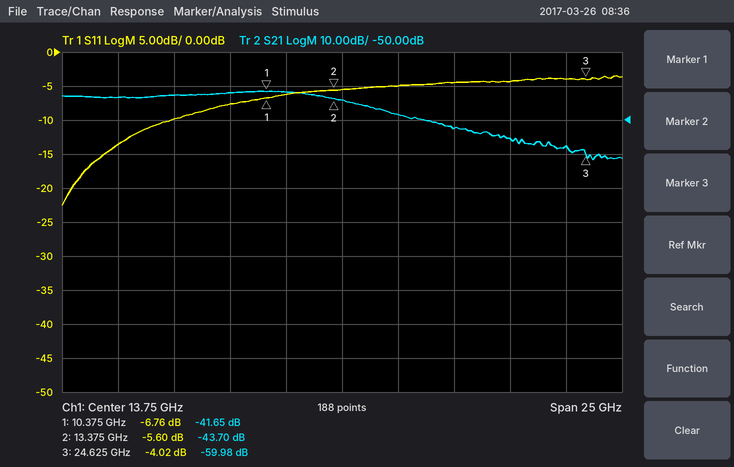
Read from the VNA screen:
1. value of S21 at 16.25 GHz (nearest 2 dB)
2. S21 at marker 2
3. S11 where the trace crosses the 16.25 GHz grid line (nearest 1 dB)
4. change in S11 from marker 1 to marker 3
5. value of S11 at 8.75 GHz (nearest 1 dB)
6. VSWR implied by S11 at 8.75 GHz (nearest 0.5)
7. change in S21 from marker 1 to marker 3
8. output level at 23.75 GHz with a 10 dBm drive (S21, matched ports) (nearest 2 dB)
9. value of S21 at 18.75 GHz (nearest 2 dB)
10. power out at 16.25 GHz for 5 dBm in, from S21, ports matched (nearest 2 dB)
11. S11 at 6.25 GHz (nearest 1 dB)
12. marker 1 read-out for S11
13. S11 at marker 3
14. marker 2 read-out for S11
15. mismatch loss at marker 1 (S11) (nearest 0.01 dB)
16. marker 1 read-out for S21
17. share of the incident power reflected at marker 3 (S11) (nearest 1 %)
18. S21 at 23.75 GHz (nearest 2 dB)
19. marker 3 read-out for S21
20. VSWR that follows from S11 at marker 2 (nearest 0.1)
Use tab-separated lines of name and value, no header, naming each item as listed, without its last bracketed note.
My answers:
value of S21 at 16.25 GHz	-48 dB
S21 at marker 2	-43.70 dB
S11 where the trace crosses the 16.25 GHz grid line	-5 dB
change in S11 from marker 1 to marker 3	2.74 dB
value of S11 at 8.75 GHz	-8 dB
VSWR implied by S11 at 8.75 GHz	2.5
change in S21 from marker 1 to marker 3	-18.33 dB
output level at 23.75 GHz with a 10 dBm drive (S21, matched ports)	-48 dBm
value of S21 at 18.75 GHz	-52 dB
power out at 16.25 GHz for 5 dBm in, from S21, ports matched	-44 dBm
S11 at 6.25 GHz	-10 dB
marker 1 read-out for S11	-6.76 dB
S11 at marker 3	-4.02 dB
marker 2 read-out for S11	-5.60 dB
mismatch loss at marker 1 (S11)	1.03 dB
marker 1 read-out for S21	-41.65 dB
share of the incident power reflected at marker 3 (S11)	40 %
S21 at 23.75 GHz	-58 dB
marker 3 read-out for S21	-59.98 dB
VSWR that follows from S11 at marker 2	3.2
